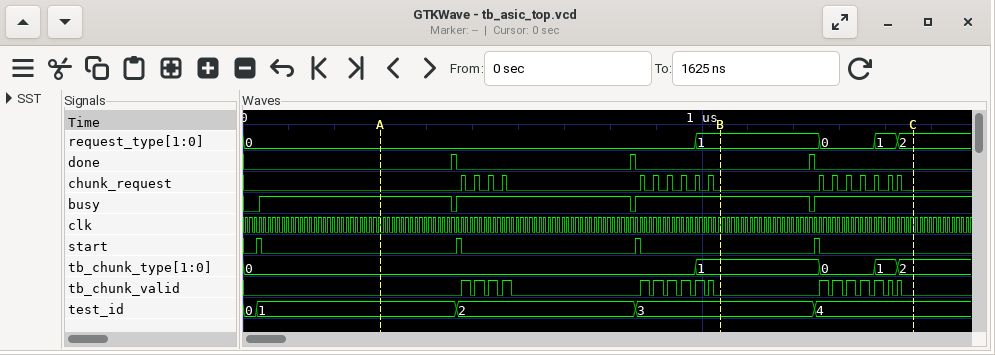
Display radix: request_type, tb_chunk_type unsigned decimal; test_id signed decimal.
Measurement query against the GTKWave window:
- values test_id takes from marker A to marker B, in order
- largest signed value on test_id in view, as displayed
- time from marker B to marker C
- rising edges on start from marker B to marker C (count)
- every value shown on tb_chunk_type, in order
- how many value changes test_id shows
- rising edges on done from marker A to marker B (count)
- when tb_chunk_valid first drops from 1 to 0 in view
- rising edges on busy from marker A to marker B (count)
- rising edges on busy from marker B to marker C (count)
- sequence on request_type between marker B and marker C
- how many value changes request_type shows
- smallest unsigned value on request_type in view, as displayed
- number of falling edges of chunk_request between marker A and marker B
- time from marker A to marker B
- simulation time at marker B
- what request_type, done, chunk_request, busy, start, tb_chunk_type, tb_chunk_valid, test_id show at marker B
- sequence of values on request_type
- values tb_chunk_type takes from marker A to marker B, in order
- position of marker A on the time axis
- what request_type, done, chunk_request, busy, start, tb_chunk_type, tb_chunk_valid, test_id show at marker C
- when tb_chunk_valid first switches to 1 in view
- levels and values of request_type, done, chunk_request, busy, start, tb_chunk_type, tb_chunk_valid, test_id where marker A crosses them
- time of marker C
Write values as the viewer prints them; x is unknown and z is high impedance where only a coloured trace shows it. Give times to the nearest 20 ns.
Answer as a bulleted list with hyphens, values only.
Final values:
- 1, 2, 3
- 4
- 420 ns
- 1
- 0, 1, 0, 1, 2
- 4
- 2
- 500 ns
- 2
- 1
- 1, 0, 1, 2
- 4
- 0
- 10
- 740 ns
- 1040 ns
- request_type=1, done=0, chunk_request=0, busy=1, start=0, tb_chunk_type=1, tb_chunk_valid=0, test_id=3
- 0, 1, 0, 1, 2
- 0, 1
- 300 ns
- request_type=2, done=0, chunk_request=0, busy=1, start=0, tb_chunk_type=2, tb_chunk_valid=0, test_id=4
- 480 ns
- request_type=0, done=0, chunk_request=0, busy=1, start=0, tb_chunk_type=0, tb_chunk_valid=0, test_id=1
- 1460 ns
